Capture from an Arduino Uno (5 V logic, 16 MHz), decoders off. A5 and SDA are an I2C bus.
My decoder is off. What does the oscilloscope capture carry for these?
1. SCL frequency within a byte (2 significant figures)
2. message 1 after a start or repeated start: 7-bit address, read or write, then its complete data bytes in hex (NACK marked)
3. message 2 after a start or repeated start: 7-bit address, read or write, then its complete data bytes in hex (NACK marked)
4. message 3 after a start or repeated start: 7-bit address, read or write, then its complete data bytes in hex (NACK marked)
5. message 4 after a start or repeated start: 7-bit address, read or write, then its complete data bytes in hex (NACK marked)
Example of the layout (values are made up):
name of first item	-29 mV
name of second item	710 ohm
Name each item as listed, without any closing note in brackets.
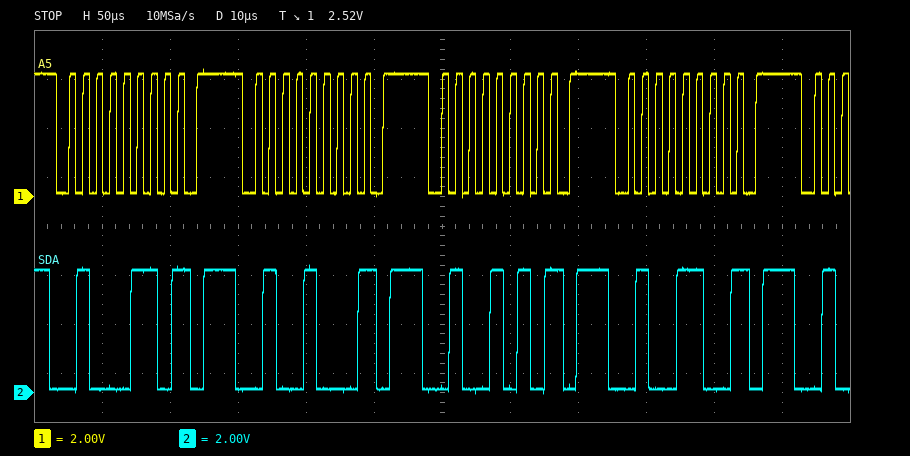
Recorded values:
SCL frequency within a byte	100 kHz
message 1 after a start or repeated start: 7-bit address, read or write, then its complete data bytes in hex	0x23 write NACK
message 2 after a start or repeated start: 7-bit address, read or write, then its complete data bytes in hex	0x24 write NACK
message 3 after a start or repeated start: 7-bit address, read or write, then its complete data bytes in hex	0x25 write NACK
message 4 after a start or repeated start: 7-bit address, read or write, then its complete data bytes in hex	0x26 write NACK
